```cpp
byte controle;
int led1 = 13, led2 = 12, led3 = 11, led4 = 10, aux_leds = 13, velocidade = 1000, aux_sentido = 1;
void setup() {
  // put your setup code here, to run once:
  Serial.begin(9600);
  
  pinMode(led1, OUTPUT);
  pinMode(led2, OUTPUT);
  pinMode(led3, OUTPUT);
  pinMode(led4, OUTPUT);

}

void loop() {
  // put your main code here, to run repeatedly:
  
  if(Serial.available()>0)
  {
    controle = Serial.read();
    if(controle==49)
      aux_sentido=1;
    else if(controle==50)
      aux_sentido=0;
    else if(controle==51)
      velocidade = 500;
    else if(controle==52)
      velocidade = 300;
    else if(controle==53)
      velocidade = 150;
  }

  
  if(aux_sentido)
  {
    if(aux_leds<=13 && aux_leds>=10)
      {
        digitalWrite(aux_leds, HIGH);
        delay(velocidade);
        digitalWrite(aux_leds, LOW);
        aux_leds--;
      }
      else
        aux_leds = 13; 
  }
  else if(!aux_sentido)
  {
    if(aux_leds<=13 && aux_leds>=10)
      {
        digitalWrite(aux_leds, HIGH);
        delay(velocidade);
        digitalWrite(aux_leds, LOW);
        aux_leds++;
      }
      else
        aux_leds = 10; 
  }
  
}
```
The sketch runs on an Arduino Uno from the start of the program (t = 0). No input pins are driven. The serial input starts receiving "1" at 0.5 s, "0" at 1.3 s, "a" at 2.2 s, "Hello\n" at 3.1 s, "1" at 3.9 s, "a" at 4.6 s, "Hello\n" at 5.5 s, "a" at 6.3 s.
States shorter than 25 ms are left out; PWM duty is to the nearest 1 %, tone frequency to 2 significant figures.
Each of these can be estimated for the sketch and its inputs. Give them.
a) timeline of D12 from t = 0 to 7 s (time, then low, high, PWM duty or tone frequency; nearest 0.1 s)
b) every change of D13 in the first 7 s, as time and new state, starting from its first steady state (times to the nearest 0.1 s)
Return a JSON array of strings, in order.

["0 s low; 1 s high; 2 s low; 5 s high; 6 s low", "0 s high; 1 s low; 4 s high; 5 s low"]
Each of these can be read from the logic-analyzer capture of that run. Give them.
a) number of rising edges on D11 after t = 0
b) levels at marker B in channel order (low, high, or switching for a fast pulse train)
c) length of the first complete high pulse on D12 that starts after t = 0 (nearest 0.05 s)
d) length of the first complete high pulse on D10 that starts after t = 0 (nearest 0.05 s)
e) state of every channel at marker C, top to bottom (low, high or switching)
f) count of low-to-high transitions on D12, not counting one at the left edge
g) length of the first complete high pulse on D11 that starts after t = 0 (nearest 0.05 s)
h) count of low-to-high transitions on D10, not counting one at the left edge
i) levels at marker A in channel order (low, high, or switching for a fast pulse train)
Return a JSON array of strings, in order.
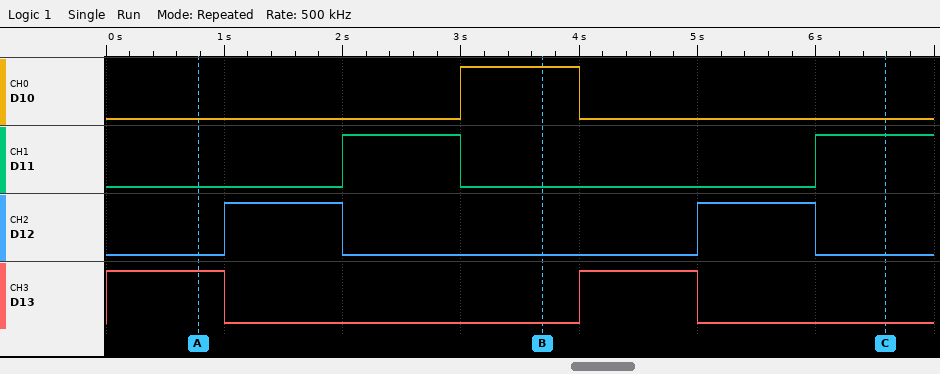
["2", "D10 high, D11 low, D12 low, D13 low", "1.00 s", "1.00 s", "D10 low, D11 high, D12 low, D13 low", "2", "1.00 s", "1", "D10 low, D11 low, D12 low, D13 high"]
